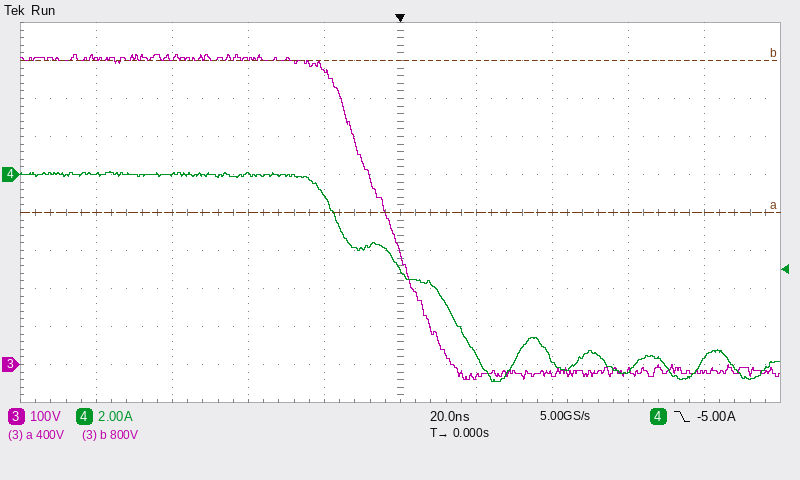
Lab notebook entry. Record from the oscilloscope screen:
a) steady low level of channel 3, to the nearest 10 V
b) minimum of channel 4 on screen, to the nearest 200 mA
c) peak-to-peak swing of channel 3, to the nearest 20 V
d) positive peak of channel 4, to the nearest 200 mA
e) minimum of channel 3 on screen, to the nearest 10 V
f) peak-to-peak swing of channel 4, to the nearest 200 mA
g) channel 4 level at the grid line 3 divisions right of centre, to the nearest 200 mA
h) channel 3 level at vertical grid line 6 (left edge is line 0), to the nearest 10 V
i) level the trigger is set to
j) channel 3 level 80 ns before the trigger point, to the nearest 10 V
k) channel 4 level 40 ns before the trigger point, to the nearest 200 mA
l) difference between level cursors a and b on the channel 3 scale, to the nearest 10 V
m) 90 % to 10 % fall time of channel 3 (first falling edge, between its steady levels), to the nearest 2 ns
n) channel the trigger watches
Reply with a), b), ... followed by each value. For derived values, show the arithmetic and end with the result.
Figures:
a) -20 V
b) -10.8 A
c) 860 V
d) 200 mA
e) -40 V
f) 200 mA − (-10.8 A) = 11.0 A
g) -10.4 A
h) -30 V
i) -5.00 A
j) 810 V
k) 0.0 A
l) 400 V
m) 26 ns
n) channel 4
